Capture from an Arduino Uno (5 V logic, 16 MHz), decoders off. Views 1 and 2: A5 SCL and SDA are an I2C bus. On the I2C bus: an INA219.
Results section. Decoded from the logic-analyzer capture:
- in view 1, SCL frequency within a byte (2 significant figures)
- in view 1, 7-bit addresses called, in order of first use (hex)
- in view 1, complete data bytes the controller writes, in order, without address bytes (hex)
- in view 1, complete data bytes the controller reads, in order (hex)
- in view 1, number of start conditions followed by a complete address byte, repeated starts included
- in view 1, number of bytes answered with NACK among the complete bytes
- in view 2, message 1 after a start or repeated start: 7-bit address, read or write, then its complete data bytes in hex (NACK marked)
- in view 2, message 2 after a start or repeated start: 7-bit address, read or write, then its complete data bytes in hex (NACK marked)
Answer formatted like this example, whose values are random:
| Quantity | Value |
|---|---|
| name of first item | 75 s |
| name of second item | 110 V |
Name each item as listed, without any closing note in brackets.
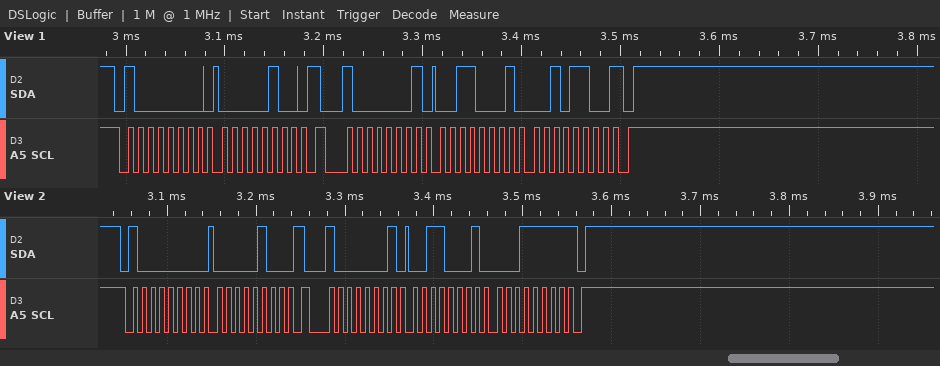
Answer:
| Quantity | Value |
|---|---|
| in view 1, SCL frequency within a byte | 100 kHz |
| in view 1, 7-bit addresses called, in order of first use | 0x40 |
| in view 1, complete data bytes the controller writes, in order, without address bytes | 04 |
| in view 1, complete data bytes the controller reads, in order | 31 2C |
| in view 1, number of start conditions followed by a complete address byte, repeated starts included | 2 |
| in view 1, number of bytes answered with NACK among the complete bytes | 1 |
| in view 2, message 1 after a start or repeated start: 7-bit address, read or write, then its complete data bytes in hex | 0x40 write: 04 |
| in view 2, message 2 after a start or repeated start: 7-bit address, read or write, then its complete data bytes in hex | 0x40 read: 31 1F NACK |
